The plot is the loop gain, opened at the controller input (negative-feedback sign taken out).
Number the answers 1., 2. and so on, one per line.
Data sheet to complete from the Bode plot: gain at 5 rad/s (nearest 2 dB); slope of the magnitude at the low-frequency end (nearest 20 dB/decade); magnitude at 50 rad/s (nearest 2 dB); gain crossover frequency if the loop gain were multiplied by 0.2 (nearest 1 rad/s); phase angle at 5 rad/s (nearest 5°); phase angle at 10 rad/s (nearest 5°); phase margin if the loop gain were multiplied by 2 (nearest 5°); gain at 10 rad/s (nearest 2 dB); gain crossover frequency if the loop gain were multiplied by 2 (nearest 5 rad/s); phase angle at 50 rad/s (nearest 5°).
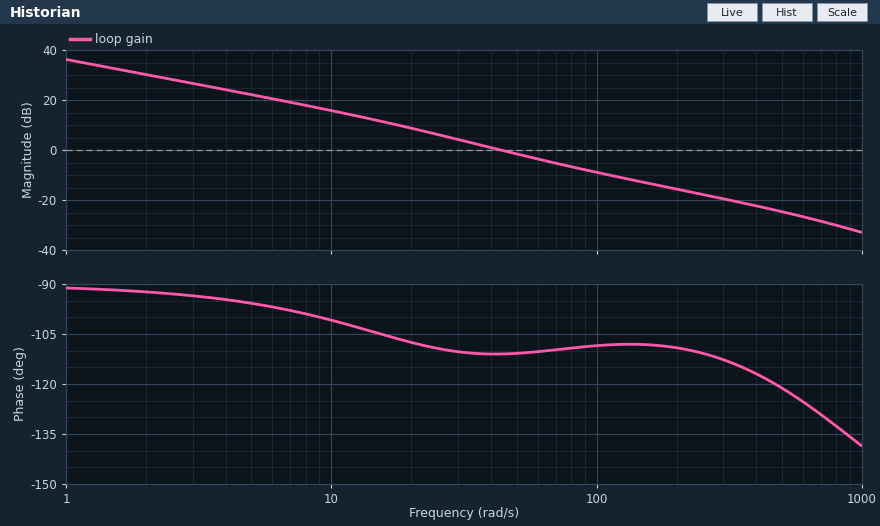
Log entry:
1. 22 dB
2. -20 dB/decade
3. -2 dB
4. 12 rad/s
5. -95°
6. -100°
7. 70°
8. 16 dB
9. 75 rad/s
10. -110°
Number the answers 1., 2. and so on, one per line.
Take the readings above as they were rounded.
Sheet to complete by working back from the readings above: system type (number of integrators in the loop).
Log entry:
1. 1
